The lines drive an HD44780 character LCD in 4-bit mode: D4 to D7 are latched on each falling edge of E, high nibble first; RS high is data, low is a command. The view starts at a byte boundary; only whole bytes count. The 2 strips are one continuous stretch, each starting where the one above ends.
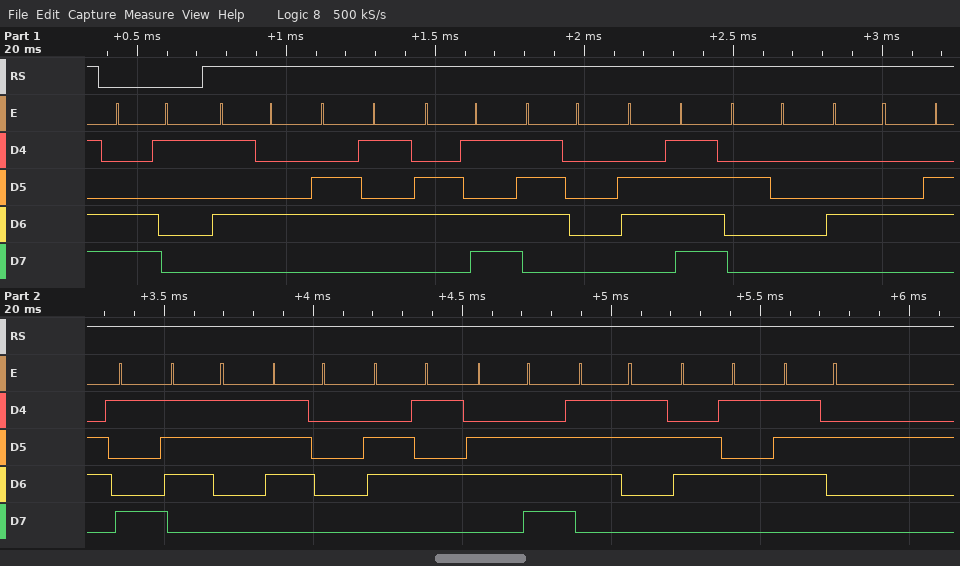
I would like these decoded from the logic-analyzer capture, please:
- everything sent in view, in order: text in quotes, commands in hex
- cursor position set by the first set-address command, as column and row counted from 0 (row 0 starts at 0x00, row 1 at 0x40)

0xC1 "Tempo Dispenser"
column 1, row 1
